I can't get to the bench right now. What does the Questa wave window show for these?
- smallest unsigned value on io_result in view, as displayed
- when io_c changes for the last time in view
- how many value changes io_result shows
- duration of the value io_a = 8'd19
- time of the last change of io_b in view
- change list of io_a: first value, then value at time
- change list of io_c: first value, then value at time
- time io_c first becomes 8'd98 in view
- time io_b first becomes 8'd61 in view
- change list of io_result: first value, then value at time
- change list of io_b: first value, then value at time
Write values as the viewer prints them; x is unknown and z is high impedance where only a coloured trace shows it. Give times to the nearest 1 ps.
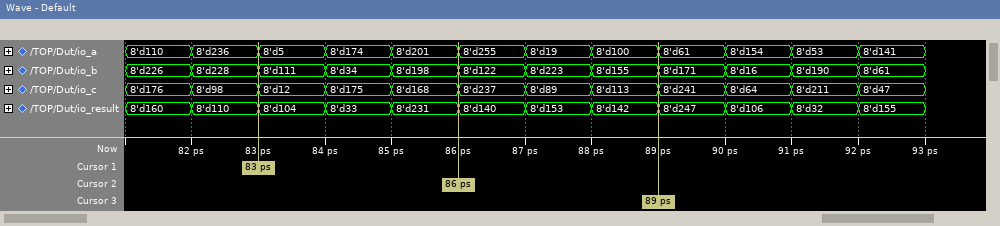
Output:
8'd32
92 ps
11
1 ps
92 ps
8'd110, 8'd236 at 82 ps, 8'd5 at 83 ps, 8'd174 at 84 ps, 8'd201 at 85 ps, 8'd255 at 86 ps, 8'd19 at 87 ps, 8'd100 at 88 ps, 8'd61 at 89 ps, 8'd154 at 90 ps, 8'd53 at 91 ps, 8'd141 at 92 ps
8'd176, 8'd98 at 82 ps, 8'd12 at 83 ps, 8'd175 at 84 ps, 8'd168 at 85 ps, 8'd237 at 86 ps, 8'd89 at 87 ps, 8'd113 at 88 ps, 8'd241 at 89 ps, 8'd64 at 90 ps, 8'd211 at 91 ps, 8'd47 at 92 ps
82 ps
92 ps
8'd160, 8'd110 at 82 ps, 8'd104 at 83 ps, 8'd33 at 84 ps, 8'd231 at 85 ps, 8'd140 at 86 ps, 8'd153 at 87 ps, 8'd142 at 88 ps, 8'd247 at 89 ps, 8'd106 at 90 ps, 8'd32 at 91 ps, 8'd155 at 92 ps
8'd226, 8'd228 at 82 ps, 8'd111 at 83 ps, 8'd34 at 84 ps, 8'd198 at 85 ps, 8'd122 at 86 ps, 8'd223 at 87 ps, 8'd155 at 88 ps, 8'd171 at 89 ps, 8'd16 at 90 ps, 8'd190 at 91 ps, 8'd61 at 92 ps
